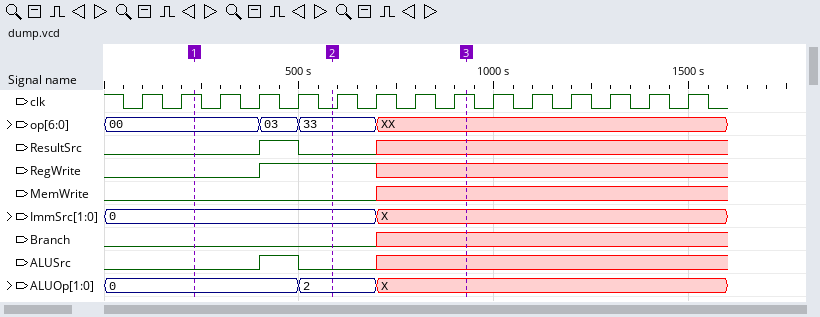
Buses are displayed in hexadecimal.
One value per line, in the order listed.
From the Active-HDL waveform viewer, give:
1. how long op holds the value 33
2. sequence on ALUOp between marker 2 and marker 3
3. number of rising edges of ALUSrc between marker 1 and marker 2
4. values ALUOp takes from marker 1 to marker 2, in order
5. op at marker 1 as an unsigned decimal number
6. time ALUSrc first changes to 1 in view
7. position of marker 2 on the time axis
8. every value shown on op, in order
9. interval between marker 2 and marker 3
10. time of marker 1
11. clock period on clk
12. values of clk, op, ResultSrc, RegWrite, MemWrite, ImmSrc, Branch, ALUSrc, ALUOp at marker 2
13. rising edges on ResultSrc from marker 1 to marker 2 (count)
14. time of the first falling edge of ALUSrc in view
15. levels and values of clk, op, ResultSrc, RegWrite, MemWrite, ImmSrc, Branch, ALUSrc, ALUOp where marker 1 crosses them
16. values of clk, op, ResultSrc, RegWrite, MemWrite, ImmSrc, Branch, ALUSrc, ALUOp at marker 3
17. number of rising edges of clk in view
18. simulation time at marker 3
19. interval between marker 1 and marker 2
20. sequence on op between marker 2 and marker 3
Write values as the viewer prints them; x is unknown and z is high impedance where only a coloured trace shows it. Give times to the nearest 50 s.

200 s
2, X
1
0, 2
0
400 s
600 s
00, 03, 33, XX
350 s
250 s
100 s
clk=0, op=33, ResultSrc=0, RegWrite=1, MemWrite=0, ImmSrc=0, Branch=0, ALUSrc=0, ALUOp=2
1
500 s
clk=1, op=00, ResultSrc=0, RegWrite=0, MemWrite=0, ImmSrc=0, Branch=0, ALUSrc=0, ALUOp=0
clk=1, op=XX, ResultSrc=x, RegWrite=x, MemWrite=x, ImmSrc=X, Branch=x, ALUSrc=x, ALUOp=X
15
950 s
350 s
33, XX
